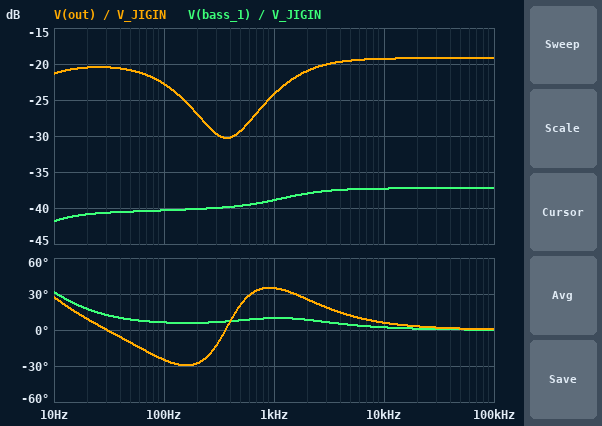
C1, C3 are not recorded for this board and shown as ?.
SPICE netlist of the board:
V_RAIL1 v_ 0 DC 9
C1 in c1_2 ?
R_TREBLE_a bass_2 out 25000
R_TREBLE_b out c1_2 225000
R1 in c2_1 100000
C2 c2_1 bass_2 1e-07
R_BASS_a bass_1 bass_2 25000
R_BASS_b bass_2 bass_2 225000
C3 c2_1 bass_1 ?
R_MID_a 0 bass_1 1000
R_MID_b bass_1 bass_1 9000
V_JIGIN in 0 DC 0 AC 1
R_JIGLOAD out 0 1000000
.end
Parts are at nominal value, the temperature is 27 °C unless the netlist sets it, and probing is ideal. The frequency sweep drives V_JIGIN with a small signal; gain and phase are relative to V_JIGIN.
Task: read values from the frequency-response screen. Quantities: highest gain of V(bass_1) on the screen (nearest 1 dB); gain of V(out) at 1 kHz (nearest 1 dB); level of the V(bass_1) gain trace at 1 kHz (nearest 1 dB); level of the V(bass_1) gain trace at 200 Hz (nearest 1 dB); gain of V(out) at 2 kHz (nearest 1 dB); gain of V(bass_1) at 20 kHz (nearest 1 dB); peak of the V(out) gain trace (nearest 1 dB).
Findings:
-37 dB
-24 dB
-39 dB
-40 dB
-21 dB
-37 dB
-19 dB
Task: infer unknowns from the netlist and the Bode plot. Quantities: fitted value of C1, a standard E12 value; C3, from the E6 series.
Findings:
470 pF
150 nF
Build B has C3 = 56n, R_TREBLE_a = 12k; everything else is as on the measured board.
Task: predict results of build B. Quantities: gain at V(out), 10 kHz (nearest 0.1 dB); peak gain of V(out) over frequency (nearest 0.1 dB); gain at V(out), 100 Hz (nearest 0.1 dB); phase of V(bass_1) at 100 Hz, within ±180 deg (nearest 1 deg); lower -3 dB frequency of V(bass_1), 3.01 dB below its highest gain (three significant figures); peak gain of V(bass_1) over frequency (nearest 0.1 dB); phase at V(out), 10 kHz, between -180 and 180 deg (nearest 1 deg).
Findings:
-24.1 dB
-17.0 dB
-17.6 dB
9 deg
364 Hz
-37.1 dB
3 deg
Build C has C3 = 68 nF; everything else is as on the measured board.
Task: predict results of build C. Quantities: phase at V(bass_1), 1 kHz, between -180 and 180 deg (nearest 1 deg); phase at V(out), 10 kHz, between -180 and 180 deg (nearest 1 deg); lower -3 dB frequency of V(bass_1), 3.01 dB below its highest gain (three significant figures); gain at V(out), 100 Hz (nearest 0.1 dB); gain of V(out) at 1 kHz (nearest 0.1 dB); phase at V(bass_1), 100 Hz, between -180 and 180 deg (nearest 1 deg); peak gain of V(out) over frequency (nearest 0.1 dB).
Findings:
11 deg
5 deg
253 Hz
-18.6 dB
-24.5 dB
9 deg
-17.6 dB
